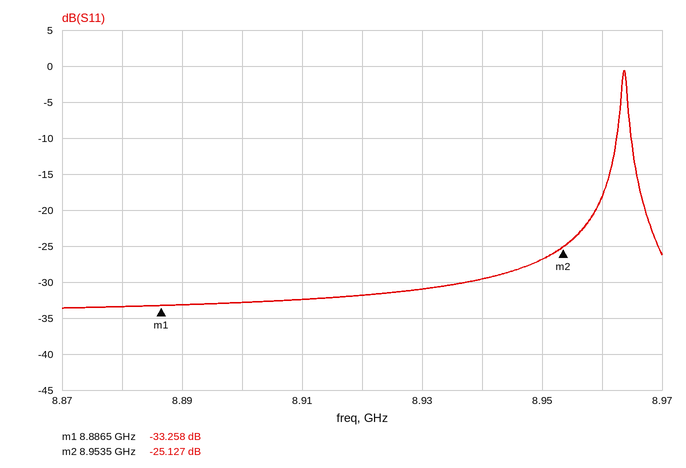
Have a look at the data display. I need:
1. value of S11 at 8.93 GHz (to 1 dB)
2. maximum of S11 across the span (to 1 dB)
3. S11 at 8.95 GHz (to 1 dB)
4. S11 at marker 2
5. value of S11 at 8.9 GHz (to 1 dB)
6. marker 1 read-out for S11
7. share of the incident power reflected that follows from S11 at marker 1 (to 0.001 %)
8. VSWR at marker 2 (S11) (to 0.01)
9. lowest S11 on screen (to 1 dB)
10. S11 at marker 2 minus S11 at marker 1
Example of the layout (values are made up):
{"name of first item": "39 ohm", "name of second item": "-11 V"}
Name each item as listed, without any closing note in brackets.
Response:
{"value of S11 at 8.93 GHz": "-31 dB", "maximum of S11 across the span": "-1 dB", "S11 at 8.95 GHz": "-27 dB", "S11 at marker 2": "-25.127 dB", "value of S11 at 8.9 GHz": "-33 dB", "marker 1 read-out for S11": "-33.258 dB", "share of the incident power reflected that follows from S11 at marker 1": "0.047 %", "VSWR at marker 2 (S11)": "1.12", "lowest S11 on screen": "-34 dB", "S11 at marker 2 minus S11 at marker 1": "8.131 dB"}
